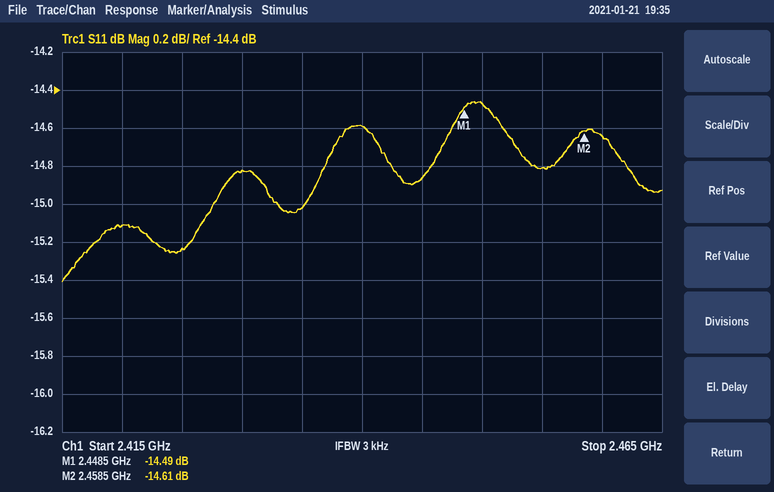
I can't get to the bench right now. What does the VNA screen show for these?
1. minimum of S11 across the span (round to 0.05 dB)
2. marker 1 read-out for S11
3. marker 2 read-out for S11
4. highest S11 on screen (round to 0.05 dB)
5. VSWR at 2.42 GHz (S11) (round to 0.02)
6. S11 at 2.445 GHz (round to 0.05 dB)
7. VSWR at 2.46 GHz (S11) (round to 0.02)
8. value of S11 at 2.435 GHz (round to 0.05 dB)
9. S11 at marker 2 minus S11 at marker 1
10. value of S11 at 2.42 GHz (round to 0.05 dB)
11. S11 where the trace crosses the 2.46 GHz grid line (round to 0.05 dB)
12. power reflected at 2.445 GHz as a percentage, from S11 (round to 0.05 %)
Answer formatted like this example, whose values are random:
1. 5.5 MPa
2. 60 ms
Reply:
1. -15.40 dB
2. -14.49 dB
3. -14.61 dB
4. -14.45 dB
5. 1.42
6. -14.85 dB
7. 1.46
8. -15.00 dB
9. -0.12 dB
10. -15.10 dB
11. -14.65 dB
12. 3.25 %
